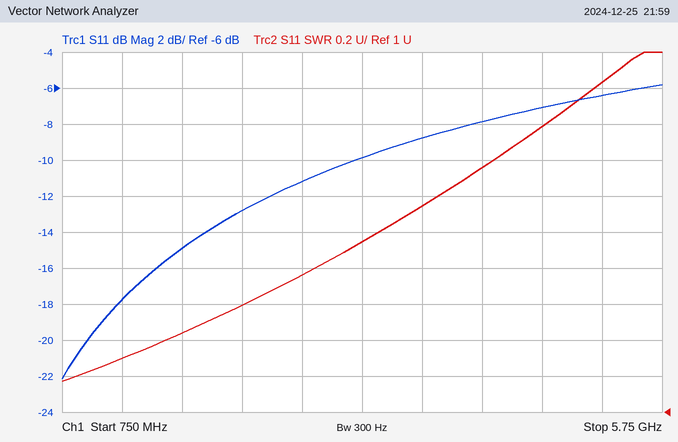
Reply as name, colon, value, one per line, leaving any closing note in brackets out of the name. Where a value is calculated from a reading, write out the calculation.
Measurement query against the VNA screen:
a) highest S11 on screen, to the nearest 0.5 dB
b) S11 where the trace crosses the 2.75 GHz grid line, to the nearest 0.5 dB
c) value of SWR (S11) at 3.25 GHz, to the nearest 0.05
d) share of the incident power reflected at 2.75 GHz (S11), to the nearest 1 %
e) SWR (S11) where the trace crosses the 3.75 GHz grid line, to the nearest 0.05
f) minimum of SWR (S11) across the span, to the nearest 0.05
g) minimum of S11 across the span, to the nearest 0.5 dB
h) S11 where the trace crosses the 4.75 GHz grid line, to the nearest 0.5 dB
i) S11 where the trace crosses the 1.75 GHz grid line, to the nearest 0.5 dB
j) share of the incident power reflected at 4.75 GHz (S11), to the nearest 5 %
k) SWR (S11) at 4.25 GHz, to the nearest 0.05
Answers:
highest S11 on screen, to the nearest 0.5 dB: -6.0 dB
S11 where the trace crosses the 2.75 GHz grid line, to the nearest 0.5 dB: -11.0 dB
value of SWR (S11) at 3.25 GHz, to the nearest 0.05: 1.95
share of the incident power reflected at 2.75 GHz (S11), to the nearest 1 %: 10^(-11/10) ≈ 8 %
SWR (S11) where the trace crosses the 3.75 GHz grid line, to the nearest 0.05: 2.15
minimum of SWR (S11) across the span, to the nearest 0.05: 1.15
minimum of S11 across the span, to the nearest 0.5 dB: -22.0 dB
S11 where the trace crosses the 4.75 GHz grid line, to the nearest 0.5 dB: -7.0 dB
S11 where the trace crosses the 1.75 GHz grid line, to the nearest 0.5 dB: -15.0 dB
share of the incident power reflected at 4.75 GHz (S11), to the nearest 5 %: 10^(-7/10) ≈ 20 %
SWR (S11) at 4.25 GHz, to the nearest 0.05: 2.35
